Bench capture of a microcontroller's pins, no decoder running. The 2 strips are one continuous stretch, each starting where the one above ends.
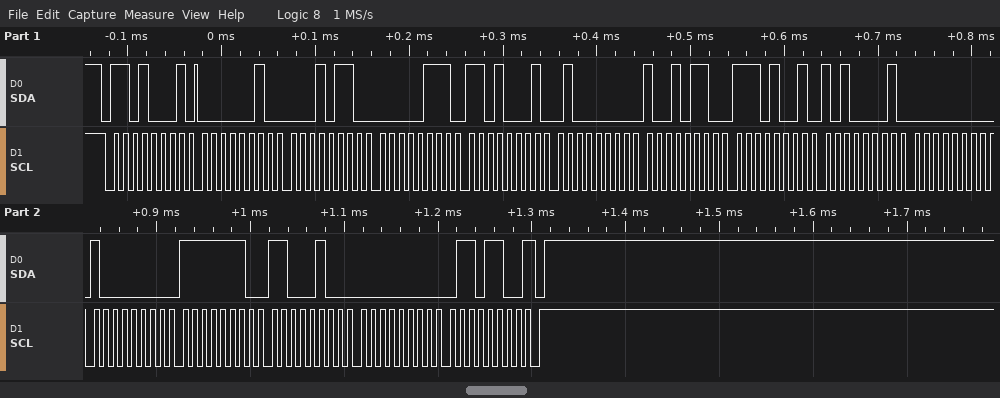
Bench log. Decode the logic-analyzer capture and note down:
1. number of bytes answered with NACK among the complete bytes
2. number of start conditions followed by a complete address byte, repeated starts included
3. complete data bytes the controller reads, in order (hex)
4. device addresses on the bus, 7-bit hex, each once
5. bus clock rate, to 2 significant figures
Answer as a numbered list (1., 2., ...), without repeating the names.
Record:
1. 1
2. 1
3. 02 16 07 D1 40 96 E9 A1 00 80 FE C4 00 6C
4. 0x68
5. 100 kHz
